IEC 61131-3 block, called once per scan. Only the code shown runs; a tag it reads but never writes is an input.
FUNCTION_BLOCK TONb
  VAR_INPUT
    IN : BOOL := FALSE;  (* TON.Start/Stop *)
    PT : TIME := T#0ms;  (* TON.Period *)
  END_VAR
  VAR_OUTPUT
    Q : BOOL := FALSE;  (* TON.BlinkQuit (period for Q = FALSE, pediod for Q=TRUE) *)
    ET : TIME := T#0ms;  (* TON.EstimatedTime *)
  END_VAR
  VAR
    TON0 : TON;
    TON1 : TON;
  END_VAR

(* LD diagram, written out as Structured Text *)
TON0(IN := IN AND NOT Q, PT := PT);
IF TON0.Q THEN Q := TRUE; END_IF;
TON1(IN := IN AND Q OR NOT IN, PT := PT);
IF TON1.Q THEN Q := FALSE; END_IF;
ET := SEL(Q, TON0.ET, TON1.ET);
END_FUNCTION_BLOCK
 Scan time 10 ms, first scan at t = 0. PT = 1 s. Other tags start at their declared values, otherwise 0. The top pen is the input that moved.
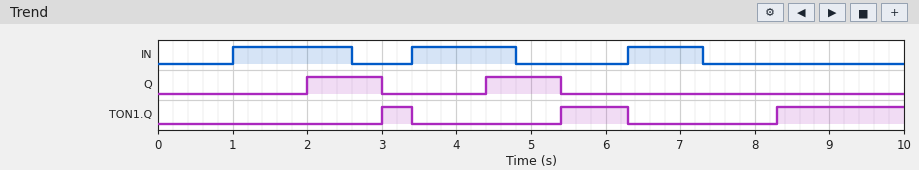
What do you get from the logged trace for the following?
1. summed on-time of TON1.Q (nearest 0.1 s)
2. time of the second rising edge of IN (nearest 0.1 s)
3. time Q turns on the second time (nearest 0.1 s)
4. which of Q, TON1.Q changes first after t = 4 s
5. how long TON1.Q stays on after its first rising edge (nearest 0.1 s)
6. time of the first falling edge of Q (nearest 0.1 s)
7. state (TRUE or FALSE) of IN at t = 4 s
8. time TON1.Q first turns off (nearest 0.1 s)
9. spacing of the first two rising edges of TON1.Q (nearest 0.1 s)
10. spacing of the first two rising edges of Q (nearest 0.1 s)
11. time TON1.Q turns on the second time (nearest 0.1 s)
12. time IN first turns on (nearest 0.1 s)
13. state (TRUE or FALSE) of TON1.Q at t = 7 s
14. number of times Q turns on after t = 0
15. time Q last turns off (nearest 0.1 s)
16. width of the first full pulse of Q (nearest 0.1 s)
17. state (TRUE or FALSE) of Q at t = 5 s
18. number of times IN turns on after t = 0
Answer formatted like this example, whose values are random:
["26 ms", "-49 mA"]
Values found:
["3.0 s", "3.4 s", "4.4 s", "Q", "0.4 s", "3.0 s", "TRUE", "3.4 s", "2.4 s", "2.4 s", "5.4 s", "1.0 s", "FALSE", "2", "5.4 s", "1.0 s", "TRUE", "3"]
